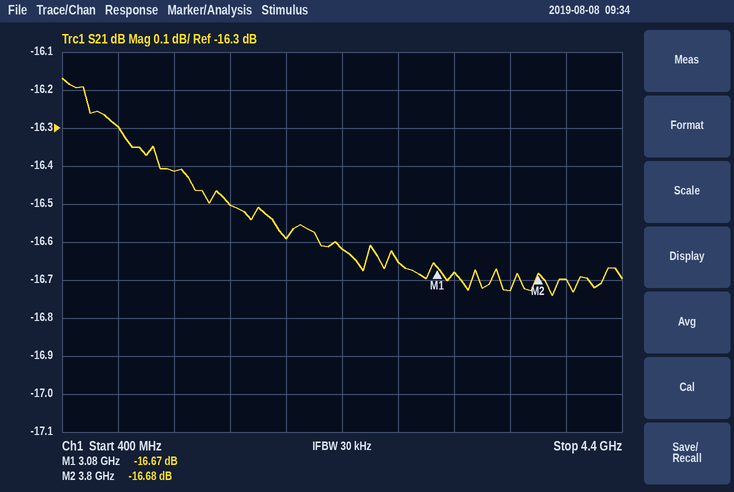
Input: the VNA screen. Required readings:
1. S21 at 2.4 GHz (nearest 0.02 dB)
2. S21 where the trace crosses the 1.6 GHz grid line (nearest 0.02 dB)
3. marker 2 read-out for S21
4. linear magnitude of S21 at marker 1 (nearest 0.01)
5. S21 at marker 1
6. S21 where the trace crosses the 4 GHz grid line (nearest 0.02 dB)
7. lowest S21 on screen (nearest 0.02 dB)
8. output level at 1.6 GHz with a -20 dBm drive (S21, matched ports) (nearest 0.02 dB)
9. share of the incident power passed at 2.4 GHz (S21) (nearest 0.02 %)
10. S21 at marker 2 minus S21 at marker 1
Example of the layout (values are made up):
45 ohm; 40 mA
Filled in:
-16.62 dB; -16.50 dB; -16.68 dB; 0.15; -16.67 dB; -16.70 dB; -16.74 dB; -36.50 dBm; 2.18 %; -0.01 dB
